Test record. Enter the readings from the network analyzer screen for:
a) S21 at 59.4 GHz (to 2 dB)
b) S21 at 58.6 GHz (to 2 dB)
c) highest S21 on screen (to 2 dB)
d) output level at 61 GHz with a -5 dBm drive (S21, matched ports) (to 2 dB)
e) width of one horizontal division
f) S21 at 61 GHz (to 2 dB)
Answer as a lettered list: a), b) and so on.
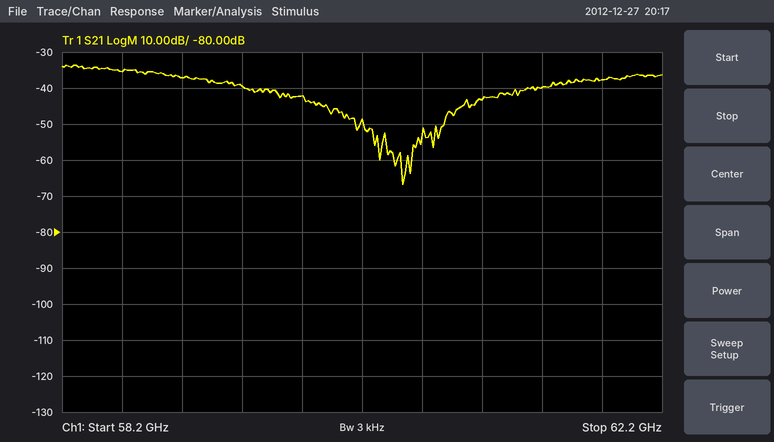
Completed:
a) -40 dB
b) -36 dB
c) -34 dB
d) -48 dBm
e) 400 MHz
f) -44 dB
